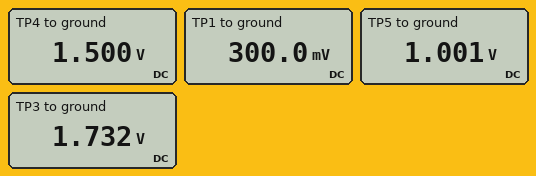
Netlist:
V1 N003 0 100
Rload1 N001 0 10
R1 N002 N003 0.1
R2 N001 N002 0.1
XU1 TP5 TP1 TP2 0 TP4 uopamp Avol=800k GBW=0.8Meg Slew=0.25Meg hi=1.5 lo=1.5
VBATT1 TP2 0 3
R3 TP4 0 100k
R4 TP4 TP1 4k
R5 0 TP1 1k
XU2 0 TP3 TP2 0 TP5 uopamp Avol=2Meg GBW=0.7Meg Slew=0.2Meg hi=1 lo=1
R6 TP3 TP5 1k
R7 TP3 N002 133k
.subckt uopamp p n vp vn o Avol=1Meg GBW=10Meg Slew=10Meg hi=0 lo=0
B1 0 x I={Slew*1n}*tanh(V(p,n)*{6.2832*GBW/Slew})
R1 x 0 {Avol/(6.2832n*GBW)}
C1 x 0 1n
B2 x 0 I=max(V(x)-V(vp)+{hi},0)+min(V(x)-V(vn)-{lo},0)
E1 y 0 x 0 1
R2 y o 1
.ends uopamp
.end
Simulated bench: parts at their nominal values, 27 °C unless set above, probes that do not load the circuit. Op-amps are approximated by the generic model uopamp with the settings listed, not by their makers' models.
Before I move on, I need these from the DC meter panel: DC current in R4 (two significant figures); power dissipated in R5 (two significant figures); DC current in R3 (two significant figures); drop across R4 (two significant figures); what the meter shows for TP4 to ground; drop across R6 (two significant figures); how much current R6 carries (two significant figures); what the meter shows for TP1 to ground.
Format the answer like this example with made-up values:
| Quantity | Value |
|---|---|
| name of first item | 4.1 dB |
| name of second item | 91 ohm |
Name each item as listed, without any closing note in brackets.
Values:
| Quantity | Value |
|---|---|
| DC current in R4 | 300 µA |
| power dissipated in R5 | 90 µW |
| DC current in R3 | 15 µA |
| drop across R4 | 1.2 V |
| what the meter shows for TP4 to ground | 1.500 V |
| drop across R6 | 730 mV |
| how much current R6 carries | 730 µA |
| what the meter shows for TP1 to ground | 300.0 mV |
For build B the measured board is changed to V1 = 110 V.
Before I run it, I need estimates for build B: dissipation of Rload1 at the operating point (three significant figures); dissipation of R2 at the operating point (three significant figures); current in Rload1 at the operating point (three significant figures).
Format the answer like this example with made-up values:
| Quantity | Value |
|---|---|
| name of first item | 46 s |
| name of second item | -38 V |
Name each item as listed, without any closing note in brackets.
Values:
| Quantity | Value |
|---|---|
| dissipation of Rload1 at the operating point | 1.16 kW |
| dissipation of R2 at the operating point | 11.6 W |
| current in Rload1 at the operating point | 10.8 A |
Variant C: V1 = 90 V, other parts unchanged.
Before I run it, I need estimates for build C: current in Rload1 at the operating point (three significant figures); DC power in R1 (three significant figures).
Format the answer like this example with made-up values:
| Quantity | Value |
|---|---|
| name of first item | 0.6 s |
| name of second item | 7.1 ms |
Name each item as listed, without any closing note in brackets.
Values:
| Quantity | Value |
|---|---|
| current in Rload1 at the operating point | 8.82 A |
| DC power in R1 | 7.79 W |
